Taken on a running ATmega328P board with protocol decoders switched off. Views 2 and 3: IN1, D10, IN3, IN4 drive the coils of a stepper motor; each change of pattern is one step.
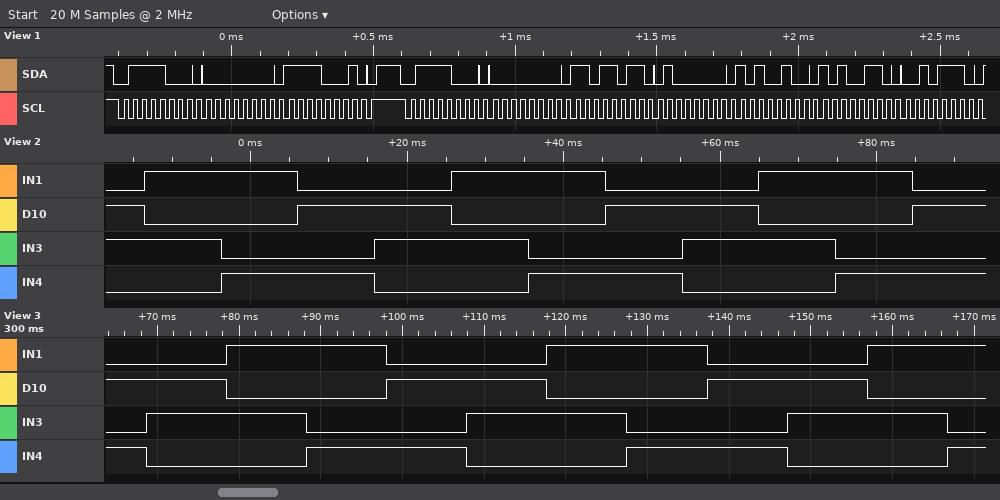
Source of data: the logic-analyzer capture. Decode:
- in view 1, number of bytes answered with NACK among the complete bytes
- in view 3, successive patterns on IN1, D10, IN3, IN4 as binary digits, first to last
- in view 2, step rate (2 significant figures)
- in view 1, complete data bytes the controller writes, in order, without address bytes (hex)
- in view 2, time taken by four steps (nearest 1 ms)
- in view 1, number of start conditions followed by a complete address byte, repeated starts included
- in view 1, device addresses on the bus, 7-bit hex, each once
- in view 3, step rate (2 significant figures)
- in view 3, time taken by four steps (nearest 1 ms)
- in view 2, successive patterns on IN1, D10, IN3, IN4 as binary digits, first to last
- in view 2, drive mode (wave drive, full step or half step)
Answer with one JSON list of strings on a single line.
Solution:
["0", "0101 0110 1010 1001 0101 0110 1010 1001 0101 0110 1010 1001", "100 steps/s", "00 F1 00 DB 40 A4 A6 2E", "39 ms", "2", "0x3C", "100 steps/s", "39 ms", "0110 1010 1001 0101 0110 1010 1001 0101 0110 1010 1001 0101", "full step"]
